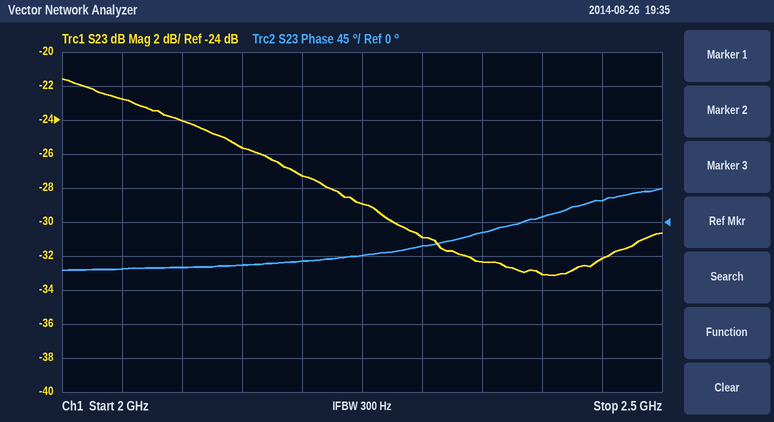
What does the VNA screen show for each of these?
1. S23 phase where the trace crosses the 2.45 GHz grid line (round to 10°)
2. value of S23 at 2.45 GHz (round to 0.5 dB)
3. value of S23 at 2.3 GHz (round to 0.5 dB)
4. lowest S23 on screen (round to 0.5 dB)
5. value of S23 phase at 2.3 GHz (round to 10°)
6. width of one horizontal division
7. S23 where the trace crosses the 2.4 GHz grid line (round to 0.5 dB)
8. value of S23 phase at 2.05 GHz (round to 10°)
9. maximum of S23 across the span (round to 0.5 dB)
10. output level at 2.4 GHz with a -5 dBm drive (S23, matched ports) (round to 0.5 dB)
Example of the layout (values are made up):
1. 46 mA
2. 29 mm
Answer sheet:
1. 30°
2. -32.0 dB
3. -31.0 dB
4. -33.0 dB
5. -30°
6. 50 MHz
7. -33.0 dB
8. -60°
9. -21.5 dB
10. -38.0 dBm
